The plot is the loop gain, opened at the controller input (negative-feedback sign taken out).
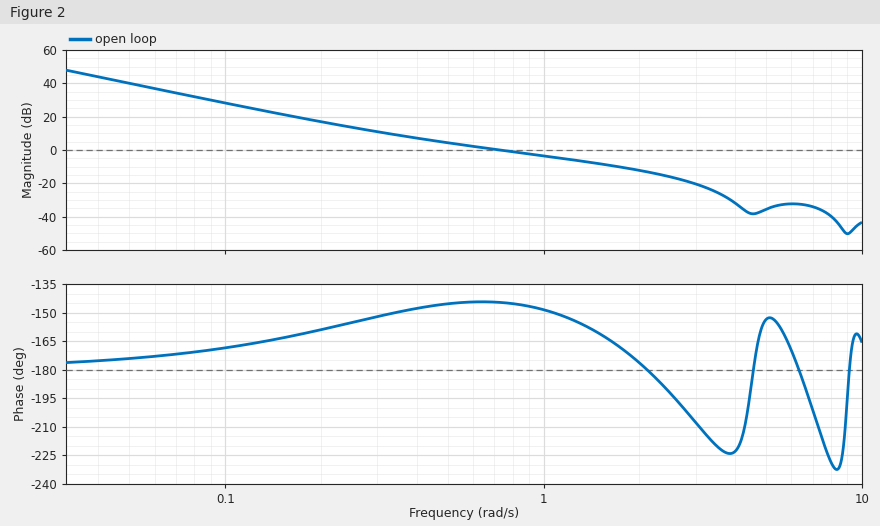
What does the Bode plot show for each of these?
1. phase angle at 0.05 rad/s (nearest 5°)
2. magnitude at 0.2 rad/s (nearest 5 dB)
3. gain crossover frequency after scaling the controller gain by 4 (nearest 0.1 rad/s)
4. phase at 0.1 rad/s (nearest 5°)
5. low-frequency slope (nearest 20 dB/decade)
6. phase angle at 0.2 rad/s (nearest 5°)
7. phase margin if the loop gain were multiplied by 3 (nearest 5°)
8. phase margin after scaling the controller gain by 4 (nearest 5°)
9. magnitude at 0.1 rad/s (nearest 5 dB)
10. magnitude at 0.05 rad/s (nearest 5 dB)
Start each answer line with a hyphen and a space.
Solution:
- -175°
- 15 dB
- 2.0 rad/s
- -170°
- -40 dB/decade
- -160°
- 15°
- 5°
- 30 dB
- 40 dB
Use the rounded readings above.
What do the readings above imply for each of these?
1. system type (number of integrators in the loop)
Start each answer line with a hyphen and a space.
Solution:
- 2
